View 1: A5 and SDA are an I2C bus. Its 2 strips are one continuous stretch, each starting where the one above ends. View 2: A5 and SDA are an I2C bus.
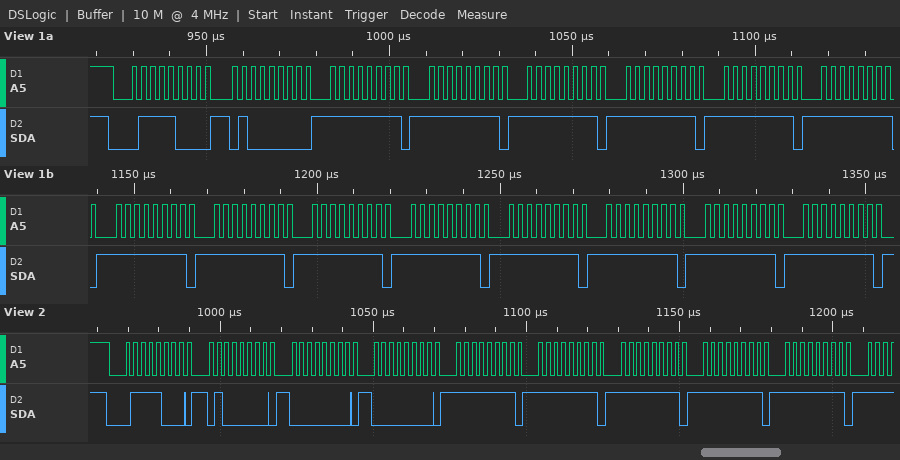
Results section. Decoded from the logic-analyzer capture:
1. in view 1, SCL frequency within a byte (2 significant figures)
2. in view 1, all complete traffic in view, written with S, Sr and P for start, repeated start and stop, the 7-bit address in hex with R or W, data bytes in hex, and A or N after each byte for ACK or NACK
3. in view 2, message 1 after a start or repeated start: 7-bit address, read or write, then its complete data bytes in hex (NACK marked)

400 kHz
S 3CW A 40 A FF A FF A FF A FF A FF A FF A FF A FF A FF A FF A FF A FF A FF A FF A
0x3C write: 40 00 00 FF FF FF FF FF
